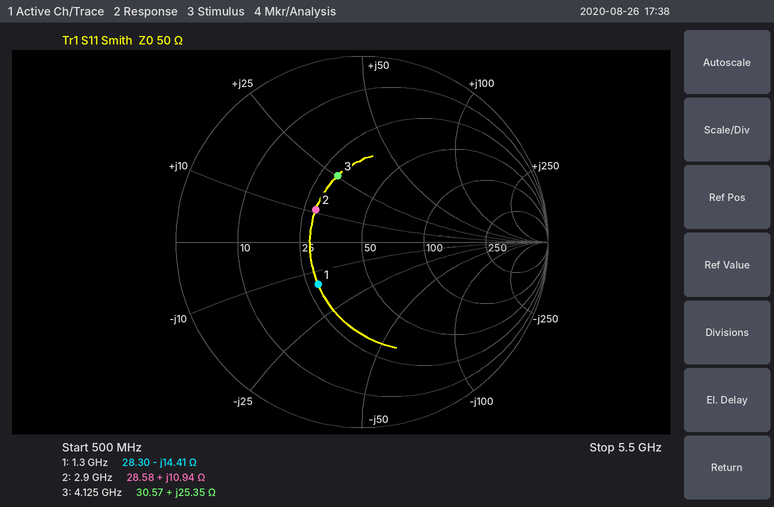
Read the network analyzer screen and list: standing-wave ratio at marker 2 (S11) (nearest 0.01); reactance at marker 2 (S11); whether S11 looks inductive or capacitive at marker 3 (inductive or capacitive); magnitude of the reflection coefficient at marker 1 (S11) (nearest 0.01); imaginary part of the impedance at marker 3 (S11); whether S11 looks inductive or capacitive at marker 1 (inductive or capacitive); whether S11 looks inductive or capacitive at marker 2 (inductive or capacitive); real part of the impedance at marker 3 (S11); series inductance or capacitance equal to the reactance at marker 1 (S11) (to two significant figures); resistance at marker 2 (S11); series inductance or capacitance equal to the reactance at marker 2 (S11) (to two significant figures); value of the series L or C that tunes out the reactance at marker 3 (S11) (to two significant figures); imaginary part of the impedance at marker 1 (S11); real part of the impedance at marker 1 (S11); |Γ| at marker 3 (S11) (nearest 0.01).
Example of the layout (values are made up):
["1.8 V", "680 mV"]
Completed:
["1.87", "+10.94 Ω", "inductive", "0.33", "+25.35 Ω", "capacitive", "inductive", "30.57 Ω", "8.5 pF", "28.58 Ω", "600 pH", "1.5 pF", "-14.41 Ω", "28.30 Ω", "0.38"]
